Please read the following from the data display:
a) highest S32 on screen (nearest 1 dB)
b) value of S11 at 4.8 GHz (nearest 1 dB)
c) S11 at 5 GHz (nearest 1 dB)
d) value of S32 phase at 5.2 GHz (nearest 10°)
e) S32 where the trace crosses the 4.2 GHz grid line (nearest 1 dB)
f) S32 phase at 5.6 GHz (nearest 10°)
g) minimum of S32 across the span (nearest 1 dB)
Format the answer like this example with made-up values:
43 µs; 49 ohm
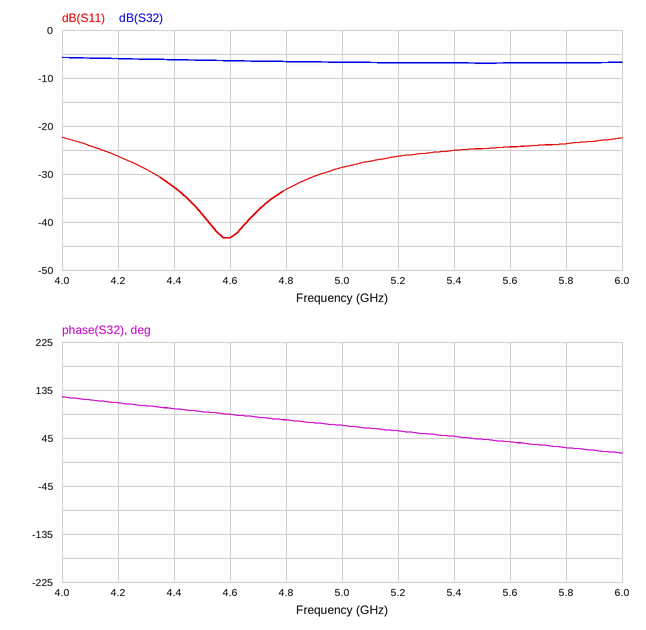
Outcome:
-6 dB; -33 dB; -29 dB; 60°; -6 dB; 40°; -7 dB
